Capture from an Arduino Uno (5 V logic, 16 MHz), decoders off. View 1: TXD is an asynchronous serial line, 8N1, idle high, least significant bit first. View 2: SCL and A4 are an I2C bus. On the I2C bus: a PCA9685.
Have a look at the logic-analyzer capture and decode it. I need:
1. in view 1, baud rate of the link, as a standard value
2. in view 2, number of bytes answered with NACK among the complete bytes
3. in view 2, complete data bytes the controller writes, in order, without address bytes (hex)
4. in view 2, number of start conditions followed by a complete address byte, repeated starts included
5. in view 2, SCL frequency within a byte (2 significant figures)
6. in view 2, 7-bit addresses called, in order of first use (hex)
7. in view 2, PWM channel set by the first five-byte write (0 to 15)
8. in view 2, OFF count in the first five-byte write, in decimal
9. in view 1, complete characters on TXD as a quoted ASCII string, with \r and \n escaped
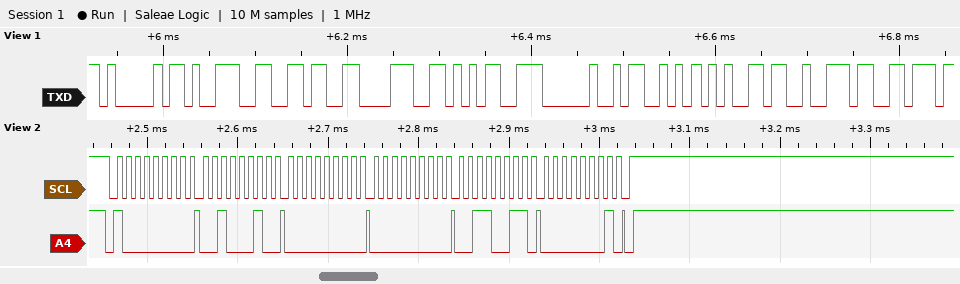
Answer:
115200 baud
0
22 00 00 33 01
1
100 kHz
0x40
7
307
"A9685 Serv"
